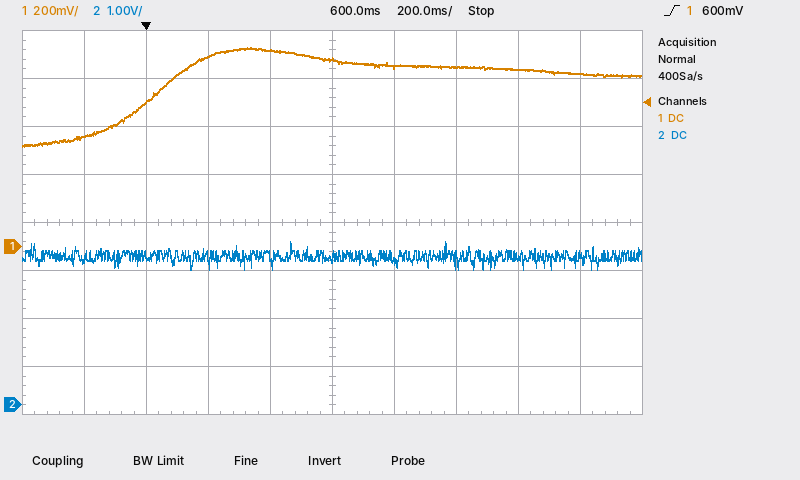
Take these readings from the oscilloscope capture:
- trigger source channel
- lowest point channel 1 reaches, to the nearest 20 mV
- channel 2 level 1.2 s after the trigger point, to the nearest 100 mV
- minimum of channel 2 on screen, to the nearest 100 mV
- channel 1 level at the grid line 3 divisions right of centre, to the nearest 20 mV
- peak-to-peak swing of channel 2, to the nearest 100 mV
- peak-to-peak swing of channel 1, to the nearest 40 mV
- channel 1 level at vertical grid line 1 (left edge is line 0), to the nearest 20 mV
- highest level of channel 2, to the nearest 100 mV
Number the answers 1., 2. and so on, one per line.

1. channel 1
2. 420 mV
3. 3.1 V
4. 2.8 V
5. 740 mV
6. 600 mV
7. 400 mV
8. 460 mV
9. 3.4 V
